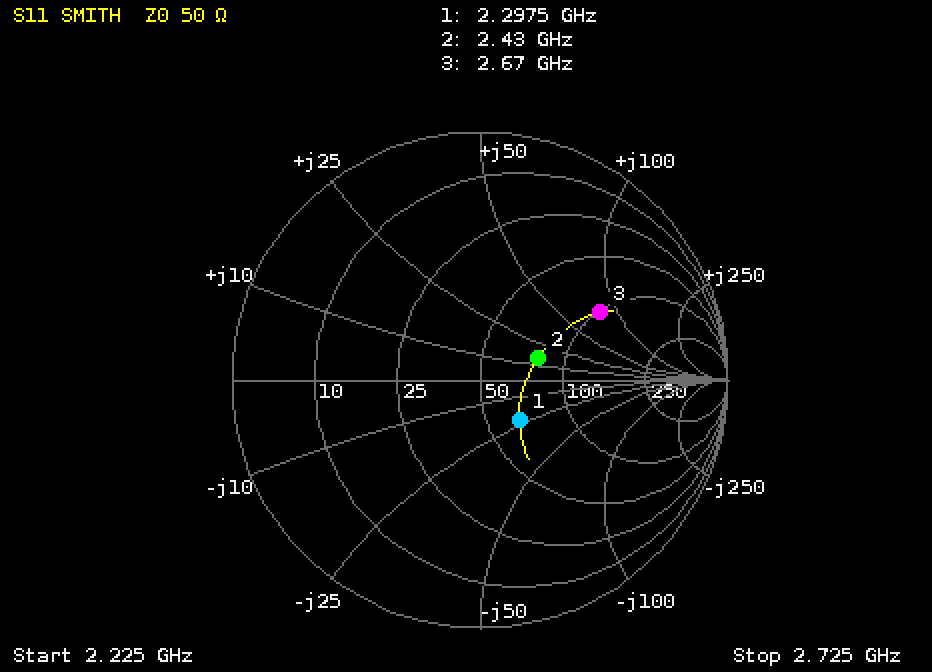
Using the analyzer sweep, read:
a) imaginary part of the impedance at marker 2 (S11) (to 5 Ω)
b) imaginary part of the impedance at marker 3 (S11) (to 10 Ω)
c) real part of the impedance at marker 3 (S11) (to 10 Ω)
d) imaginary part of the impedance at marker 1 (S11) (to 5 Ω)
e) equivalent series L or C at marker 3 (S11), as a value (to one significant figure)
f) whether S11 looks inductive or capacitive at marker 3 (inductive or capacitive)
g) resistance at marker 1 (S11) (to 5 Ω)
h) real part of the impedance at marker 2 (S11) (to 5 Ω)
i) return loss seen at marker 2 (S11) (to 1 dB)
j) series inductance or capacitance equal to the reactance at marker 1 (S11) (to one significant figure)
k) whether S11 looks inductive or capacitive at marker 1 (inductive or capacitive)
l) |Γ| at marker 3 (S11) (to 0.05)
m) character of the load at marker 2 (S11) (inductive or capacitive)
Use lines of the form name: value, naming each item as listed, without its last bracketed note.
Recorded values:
imaginary part of the impedance at marker 2 (S11): +15 Ω
imaginary part of the impedance at marker 3 (S11): +80 Ω
real part of the impedance at marker 3 (S11): 100 Ω
imaginary part of the impedance at marker 1 (S11): -20 Ω
equivalent series L or C at marker 3 (S11), as a value: 5 nH
whether S11 looks inductive or capacitive at marker 3: inductive
resistance at marker 1 (S11): 65 Ω
real part of the impedance at marker 2 (S11): 80 Ω
return loss seen at marker 2 (S11): 12 dB
series inductance or capacitance equal to the reactance at marker 1 (S11): 3 pF
whether S11 looks inductive or capacitive at marker 1: capacitive
|Γ| at marker 3 (S11): 0.55
character of the load at marker 2 (S11): inductive
